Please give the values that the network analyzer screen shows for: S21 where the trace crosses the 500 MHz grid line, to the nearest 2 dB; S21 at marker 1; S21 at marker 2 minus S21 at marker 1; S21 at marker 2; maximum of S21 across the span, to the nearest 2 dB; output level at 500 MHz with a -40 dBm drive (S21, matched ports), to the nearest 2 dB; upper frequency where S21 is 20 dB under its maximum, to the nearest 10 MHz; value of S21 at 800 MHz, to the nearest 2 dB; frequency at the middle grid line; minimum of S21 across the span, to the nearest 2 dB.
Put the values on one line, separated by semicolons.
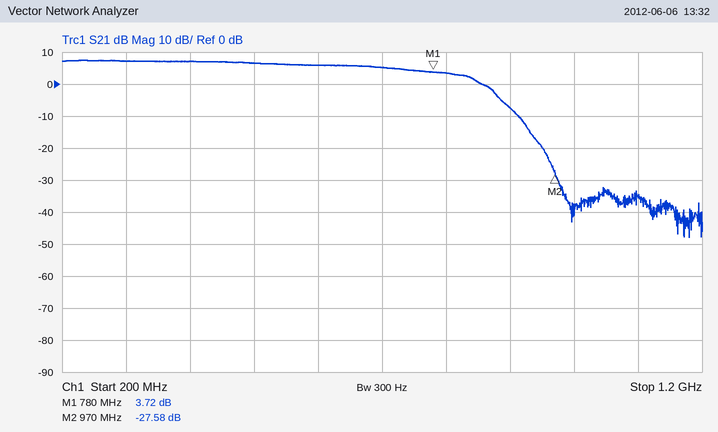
6 dB; 3.72 dB; -31.30 dB; -27.58 dB; 8 dB; -34 dBm; 920 MHz; 4 dB; 700 MHz; -48 dB
